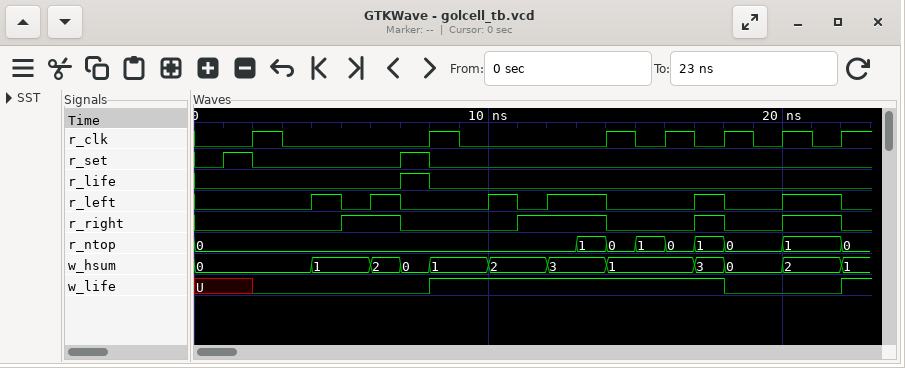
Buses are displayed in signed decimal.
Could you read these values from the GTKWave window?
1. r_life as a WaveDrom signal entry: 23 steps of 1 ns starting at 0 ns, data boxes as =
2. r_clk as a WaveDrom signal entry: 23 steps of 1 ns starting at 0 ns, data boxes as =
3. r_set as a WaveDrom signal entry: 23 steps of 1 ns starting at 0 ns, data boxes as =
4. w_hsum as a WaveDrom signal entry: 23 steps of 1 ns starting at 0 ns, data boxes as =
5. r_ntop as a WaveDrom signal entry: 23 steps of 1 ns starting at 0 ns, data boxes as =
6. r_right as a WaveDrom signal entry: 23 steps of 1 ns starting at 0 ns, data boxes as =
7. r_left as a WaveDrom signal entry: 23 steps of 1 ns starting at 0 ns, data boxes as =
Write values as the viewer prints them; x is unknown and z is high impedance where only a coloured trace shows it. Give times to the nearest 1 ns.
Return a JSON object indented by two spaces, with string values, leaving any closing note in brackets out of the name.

{
  "r_life as a WaveDrom signal entry: 23 steps of 1 ns starting at 0 ns, data boxes as =": "{name: 'r_life', wave: '0......10..............'}",
  "r_clk as a WaveDrom signal entry: 23 steps of 1 ns starting at 0 ns, data boxes as =": "{name: 'r_clk', wave: '0.10....10....101010101'}",
  "r_set as a WaveDrom signal entry: 23 steps of 1 ns starting at 0 ns, data boxes as =": "{name: 'r_set', wave: '010....10..............'}",
  "w_hsum as a WaveDrom signal entry: 23 steps of 1 ns starting at 0 ns, data boxes as =": "{name: 'w_hsum', wave: '=...=.===.=.=.=..==.=.=', data: '0 1 2 0 1 2 3 1 3 0 2 1'}",
  "r_ntop as a WaveDrom signal entry: 23 steps of 1 ns starting at 0 ns, data boxes as =": "{name: 'r_ntop', wave: '=............======.=.=', data: '0 1 0 1 0 1 0 1 0'}",
  "r_right as a WaveDrom signal entry: 23 steps of 1 ns starting at 0 ns, data boxes as =": "{name: 'r_right', wave: '0....1.0...1..0..10.1.0'}",
  "r_left as a WaveDrom signal entry: 23 steps of 1 ns starting at 0 ns, data boxes as =": "{name: 'r_left', wave: '0...1010..101.0..10.1.0'}"
}
